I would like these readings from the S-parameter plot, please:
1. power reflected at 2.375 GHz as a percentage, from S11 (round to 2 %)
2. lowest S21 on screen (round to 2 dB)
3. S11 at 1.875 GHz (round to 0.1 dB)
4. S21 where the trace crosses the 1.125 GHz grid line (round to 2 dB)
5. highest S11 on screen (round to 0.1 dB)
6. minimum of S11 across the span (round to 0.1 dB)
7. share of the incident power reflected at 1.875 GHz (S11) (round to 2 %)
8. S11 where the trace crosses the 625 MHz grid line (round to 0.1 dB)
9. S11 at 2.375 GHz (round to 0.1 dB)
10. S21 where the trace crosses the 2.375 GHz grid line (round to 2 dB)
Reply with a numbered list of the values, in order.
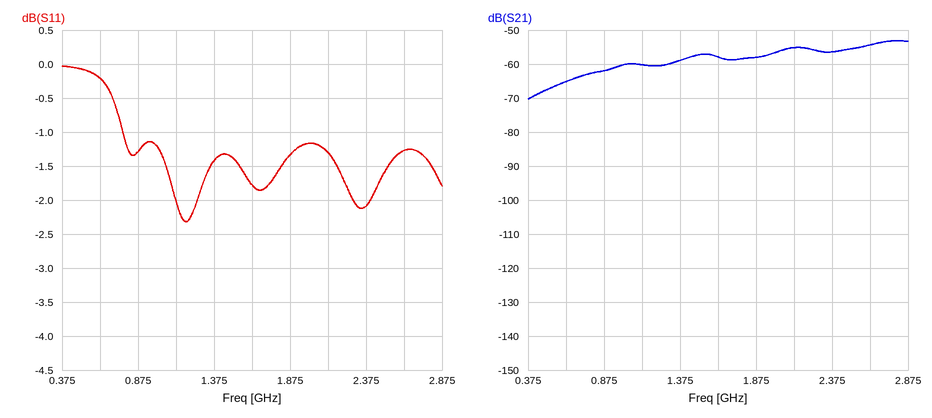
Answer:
1. 62 %
2. -70 dB
3. -1.3 dB
4. -60 dB
5. 0.0 dB
6. -2.3 dB
7. 74 %
8. -0.2 dB
9. -2.1 dB
10. -56 dB
